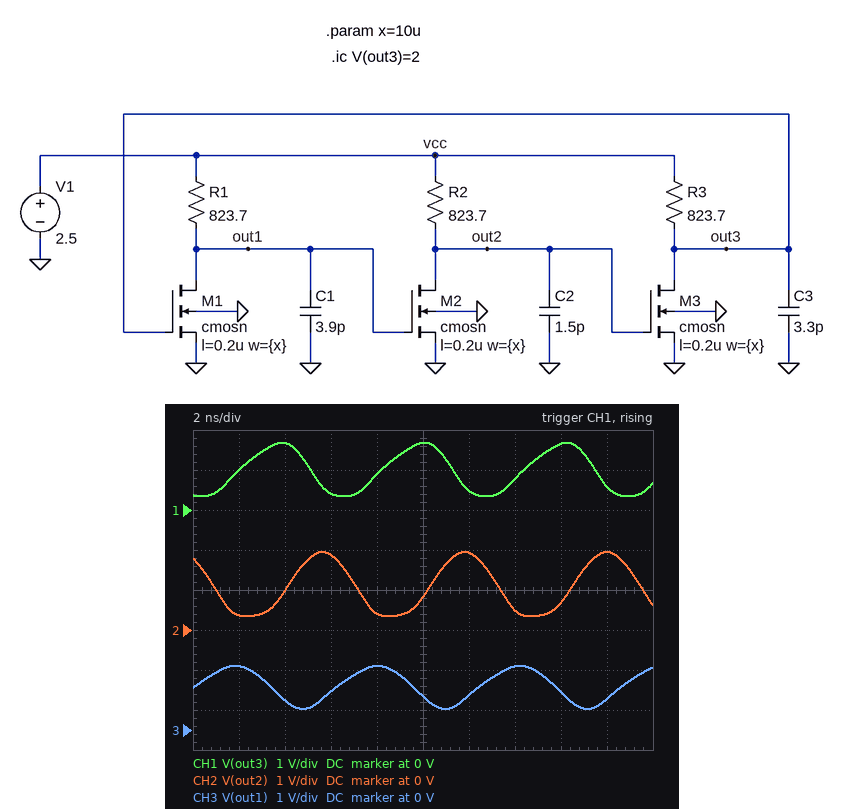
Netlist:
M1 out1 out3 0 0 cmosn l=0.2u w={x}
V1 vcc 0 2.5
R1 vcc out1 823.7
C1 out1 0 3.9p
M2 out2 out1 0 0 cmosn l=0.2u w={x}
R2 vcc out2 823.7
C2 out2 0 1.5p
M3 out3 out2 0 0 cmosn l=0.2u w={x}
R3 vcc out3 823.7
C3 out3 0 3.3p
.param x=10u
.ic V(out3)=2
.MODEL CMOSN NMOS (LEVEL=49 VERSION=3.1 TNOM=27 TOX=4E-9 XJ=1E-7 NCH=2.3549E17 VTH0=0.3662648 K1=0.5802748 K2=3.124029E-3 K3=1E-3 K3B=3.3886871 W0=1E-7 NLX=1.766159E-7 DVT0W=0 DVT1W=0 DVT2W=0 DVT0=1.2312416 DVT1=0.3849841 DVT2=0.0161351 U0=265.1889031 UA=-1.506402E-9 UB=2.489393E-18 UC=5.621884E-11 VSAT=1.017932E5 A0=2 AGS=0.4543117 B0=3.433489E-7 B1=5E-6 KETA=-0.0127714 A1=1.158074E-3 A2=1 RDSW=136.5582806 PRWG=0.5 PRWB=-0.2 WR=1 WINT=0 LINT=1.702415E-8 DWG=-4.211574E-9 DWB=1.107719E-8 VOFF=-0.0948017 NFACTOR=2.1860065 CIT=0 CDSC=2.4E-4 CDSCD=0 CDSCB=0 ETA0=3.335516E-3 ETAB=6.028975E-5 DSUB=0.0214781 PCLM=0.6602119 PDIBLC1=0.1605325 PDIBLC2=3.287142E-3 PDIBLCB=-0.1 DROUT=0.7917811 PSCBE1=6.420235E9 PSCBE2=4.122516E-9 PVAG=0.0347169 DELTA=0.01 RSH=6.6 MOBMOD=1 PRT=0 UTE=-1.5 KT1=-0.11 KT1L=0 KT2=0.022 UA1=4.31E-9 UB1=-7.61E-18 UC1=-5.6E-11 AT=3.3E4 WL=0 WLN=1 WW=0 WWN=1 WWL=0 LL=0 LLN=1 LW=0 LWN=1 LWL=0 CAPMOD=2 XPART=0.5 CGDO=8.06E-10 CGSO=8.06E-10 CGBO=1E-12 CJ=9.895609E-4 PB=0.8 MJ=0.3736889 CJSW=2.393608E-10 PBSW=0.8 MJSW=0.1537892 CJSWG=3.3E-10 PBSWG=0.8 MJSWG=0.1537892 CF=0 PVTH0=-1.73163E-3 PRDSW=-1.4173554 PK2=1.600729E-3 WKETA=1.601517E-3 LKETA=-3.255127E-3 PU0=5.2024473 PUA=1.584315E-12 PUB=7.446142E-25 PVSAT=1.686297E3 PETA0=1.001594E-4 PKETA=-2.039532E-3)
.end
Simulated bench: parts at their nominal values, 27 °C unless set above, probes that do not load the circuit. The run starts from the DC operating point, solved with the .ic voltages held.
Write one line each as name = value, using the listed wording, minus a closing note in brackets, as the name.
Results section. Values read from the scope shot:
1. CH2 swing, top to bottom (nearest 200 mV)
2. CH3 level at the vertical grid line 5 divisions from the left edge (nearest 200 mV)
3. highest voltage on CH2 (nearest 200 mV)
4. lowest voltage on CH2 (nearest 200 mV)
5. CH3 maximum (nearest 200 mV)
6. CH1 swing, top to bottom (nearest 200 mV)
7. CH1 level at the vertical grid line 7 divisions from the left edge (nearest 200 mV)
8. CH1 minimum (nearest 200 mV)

CH2 swing, top to bottom = 1.6 V
CH3 level at the vertical grid line 5 divisions from the left edge = 800 mV
highest voltage on CH2 = 2.0 V
lowest voltage on CH2 = 400 mV
CH3 maximum = 1.6 V
CH1 swing, top to bottom = 1.4 V
CH1 level at the vertical grid line 7 divisions from the left edge = 800 mV
CH1 minimum = 400 mV
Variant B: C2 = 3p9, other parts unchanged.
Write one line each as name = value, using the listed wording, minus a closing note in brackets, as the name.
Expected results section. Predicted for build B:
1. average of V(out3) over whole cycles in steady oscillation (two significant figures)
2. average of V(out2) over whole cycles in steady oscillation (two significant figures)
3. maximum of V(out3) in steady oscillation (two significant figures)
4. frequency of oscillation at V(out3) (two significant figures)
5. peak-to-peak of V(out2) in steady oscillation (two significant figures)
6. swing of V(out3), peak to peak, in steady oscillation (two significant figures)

average of V(out3) over whole cycles in steady oscillation = 1.1 V
average of V(out2) over whole cycles in steady oscillation = 1.1 V
maximum of V(out3) in steady oscillation = 1.8 V
frequency of oscillation at V(out3) = 120 MHz
peak-to-peak of V(out2) in steady oscillation = 1.4 V
swing of V(out3), peak to peak, in steady oscillation = 1.5 V
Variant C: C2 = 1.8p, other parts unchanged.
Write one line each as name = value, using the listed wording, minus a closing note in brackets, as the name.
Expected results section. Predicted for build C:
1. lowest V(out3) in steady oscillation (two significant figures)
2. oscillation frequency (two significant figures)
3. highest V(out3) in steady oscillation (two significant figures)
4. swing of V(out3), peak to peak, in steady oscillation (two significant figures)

lowest V(out3) in steady oscillation = 330 mV
oscillation frequency = 150 MHz
highest V(out3) in steady oscillation = 1.7 V
swing of V(out3), peak to peak, in steady oscillation = 1.4 V
